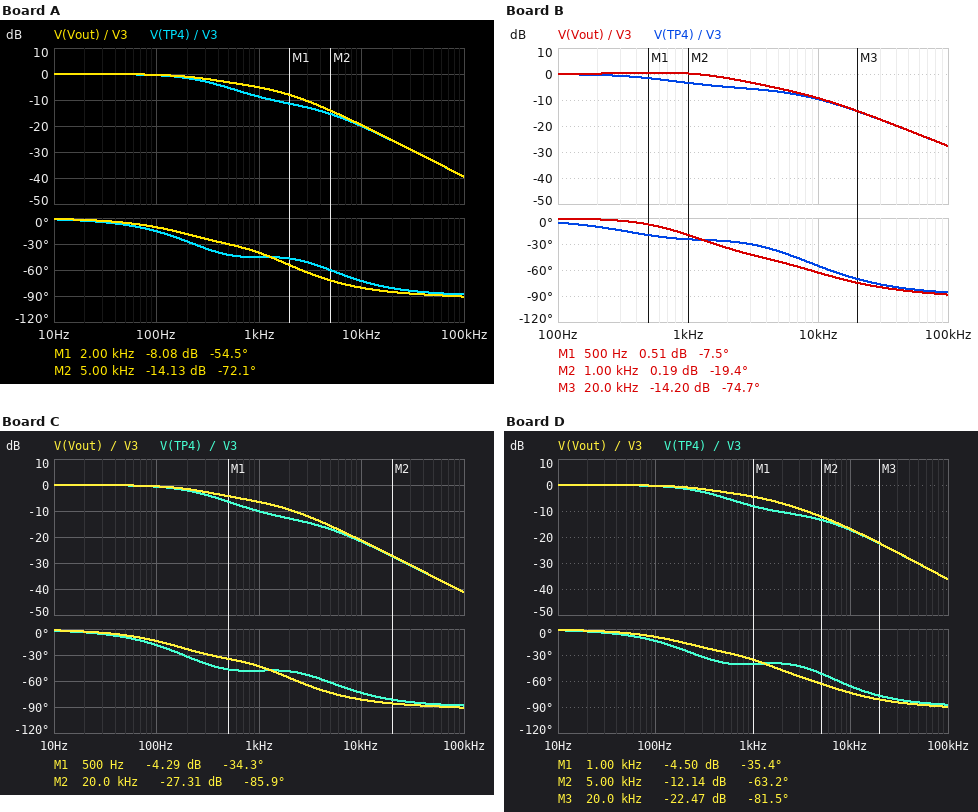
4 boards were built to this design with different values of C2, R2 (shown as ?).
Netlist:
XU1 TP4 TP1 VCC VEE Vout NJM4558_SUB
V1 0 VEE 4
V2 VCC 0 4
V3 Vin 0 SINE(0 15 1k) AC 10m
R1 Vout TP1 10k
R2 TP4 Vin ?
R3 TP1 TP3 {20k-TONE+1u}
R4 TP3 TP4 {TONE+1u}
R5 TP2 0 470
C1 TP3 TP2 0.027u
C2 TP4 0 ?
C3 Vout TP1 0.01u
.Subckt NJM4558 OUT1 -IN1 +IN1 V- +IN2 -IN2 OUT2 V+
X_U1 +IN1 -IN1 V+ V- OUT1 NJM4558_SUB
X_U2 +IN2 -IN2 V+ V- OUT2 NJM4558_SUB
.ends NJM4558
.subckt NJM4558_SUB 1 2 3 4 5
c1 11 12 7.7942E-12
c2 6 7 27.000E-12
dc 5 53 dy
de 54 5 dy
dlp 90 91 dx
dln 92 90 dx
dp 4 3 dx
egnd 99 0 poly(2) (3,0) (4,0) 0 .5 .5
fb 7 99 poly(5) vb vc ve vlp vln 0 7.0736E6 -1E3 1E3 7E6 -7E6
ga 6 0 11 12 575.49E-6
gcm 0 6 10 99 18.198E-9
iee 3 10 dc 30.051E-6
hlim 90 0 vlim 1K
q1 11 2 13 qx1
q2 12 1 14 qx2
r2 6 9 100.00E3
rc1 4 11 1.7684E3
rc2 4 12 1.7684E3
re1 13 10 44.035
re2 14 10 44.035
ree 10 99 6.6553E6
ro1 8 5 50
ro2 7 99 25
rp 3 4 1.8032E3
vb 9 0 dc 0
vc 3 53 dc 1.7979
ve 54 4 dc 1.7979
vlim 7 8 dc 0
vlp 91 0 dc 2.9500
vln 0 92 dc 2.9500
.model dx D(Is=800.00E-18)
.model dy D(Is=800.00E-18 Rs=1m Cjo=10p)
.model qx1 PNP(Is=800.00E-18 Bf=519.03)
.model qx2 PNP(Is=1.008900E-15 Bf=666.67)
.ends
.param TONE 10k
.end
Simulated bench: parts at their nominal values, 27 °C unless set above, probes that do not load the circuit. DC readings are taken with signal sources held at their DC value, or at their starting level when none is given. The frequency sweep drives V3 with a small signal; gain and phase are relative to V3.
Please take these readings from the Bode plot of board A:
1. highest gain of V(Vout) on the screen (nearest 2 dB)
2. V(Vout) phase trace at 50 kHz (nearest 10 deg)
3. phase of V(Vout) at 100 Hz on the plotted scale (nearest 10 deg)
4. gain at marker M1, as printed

0 dB
-90 deg
-10 deg
-8.08 dB
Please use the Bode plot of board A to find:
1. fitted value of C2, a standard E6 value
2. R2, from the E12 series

6.8 nF
22 kΩ
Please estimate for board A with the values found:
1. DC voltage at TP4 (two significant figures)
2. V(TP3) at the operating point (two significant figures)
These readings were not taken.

-6.1 mV
-9.1 mV
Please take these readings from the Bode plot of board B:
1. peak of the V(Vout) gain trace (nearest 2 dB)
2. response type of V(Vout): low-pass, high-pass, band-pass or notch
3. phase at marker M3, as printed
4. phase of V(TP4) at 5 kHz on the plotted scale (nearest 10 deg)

0 dB
low-pass
-74.7 deg
-40 deg
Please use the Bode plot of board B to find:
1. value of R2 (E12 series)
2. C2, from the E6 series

8.2 kΩ
4.7 nF
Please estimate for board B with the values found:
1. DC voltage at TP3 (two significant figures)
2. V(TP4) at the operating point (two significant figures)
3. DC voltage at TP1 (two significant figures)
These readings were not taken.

-5.3 mV
-2.3 mV
-8.3 mV
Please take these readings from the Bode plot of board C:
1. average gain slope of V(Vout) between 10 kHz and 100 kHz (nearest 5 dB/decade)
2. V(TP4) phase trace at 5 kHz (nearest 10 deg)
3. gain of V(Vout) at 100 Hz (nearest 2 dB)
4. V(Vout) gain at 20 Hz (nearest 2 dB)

-20 dB/decade
-60 deg
0 dB
0 dB
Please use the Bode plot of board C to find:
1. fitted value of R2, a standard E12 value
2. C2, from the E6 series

27 kΩ
6.8 nF
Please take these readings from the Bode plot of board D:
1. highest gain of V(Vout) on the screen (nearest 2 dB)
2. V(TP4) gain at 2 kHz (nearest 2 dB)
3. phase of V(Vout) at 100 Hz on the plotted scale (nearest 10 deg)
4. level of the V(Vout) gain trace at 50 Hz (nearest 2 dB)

0 dB
-10 dB
-10 deg
0 dB
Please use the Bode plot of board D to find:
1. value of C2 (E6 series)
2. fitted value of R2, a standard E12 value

4.7 nF
22 kΩ
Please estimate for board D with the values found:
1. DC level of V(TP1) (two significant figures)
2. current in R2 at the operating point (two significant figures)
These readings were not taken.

-12 mV
280 nA
